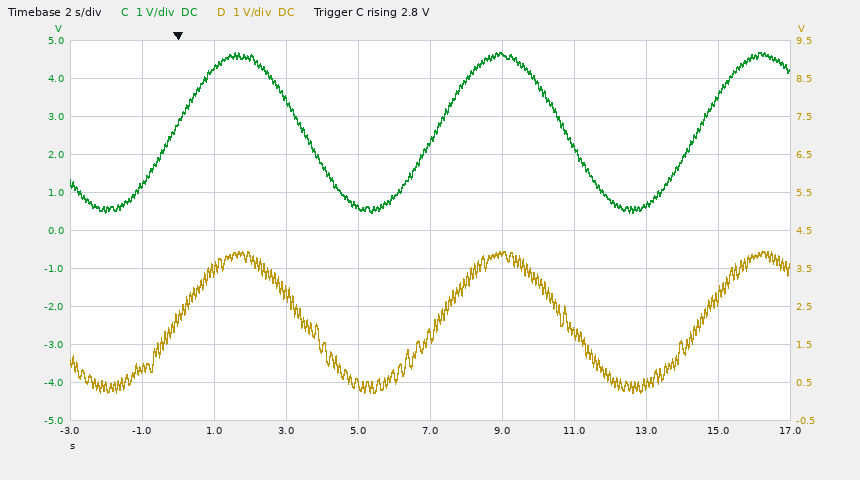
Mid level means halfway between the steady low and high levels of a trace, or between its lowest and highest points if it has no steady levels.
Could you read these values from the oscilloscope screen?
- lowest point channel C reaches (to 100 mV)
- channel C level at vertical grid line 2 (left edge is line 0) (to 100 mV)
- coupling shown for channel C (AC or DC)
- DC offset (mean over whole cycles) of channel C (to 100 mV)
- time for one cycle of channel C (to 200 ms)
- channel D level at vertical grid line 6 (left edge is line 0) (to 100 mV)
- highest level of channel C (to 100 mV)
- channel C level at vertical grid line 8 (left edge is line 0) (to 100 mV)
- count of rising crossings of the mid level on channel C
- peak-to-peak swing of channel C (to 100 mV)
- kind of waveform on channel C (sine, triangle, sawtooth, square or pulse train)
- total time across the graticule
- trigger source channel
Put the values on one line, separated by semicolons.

500 mV; 4.3 V; DC; 2.6 V; 7.2 s; 3.9 V; 4.7 V; 700 mV; 3; 4.2 V; sine; 20 s; channel C
